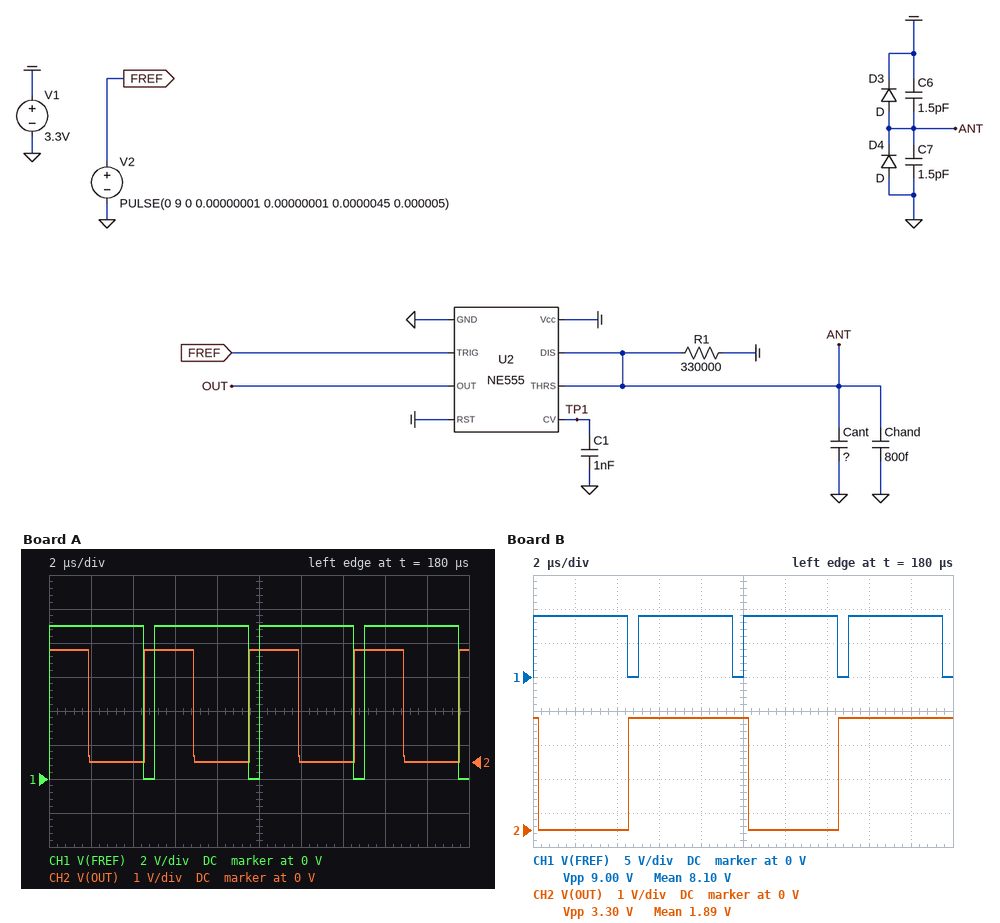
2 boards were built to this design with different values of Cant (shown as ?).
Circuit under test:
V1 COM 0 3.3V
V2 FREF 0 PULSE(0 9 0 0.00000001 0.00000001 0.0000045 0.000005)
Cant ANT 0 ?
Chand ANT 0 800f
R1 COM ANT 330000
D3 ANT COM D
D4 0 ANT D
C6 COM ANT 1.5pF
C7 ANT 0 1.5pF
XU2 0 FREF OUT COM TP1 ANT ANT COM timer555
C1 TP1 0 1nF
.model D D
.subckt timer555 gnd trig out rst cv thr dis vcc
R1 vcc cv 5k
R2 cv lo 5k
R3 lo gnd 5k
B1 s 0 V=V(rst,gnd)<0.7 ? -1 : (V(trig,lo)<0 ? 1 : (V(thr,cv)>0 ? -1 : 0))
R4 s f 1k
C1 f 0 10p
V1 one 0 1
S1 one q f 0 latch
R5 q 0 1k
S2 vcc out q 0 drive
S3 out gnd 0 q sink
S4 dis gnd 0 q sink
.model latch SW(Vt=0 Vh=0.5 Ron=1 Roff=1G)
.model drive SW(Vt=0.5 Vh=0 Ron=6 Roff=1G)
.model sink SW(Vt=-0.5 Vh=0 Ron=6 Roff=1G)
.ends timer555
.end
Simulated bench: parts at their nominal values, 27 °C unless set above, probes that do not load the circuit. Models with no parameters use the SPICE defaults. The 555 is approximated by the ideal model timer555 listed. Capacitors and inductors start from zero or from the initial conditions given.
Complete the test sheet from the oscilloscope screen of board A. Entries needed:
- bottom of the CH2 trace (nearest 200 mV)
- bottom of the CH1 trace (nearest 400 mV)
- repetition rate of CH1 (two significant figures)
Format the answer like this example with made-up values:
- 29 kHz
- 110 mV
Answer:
- 0 V
- 0 V
- 200 kHz
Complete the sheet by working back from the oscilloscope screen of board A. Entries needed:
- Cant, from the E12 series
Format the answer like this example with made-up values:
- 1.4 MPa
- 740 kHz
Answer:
- 2.7 pF
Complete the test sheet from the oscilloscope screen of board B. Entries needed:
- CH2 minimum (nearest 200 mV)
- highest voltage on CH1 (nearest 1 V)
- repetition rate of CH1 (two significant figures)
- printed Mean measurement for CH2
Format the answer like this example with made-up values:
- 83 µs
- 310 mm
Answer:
- 0 V
- 9 V
- 200 kHz
- 1.89 V
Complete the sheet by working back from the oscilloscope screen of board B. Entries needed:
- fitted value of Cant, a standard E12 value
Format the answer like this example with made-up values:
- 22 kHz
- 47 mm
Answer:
- 12 pF
